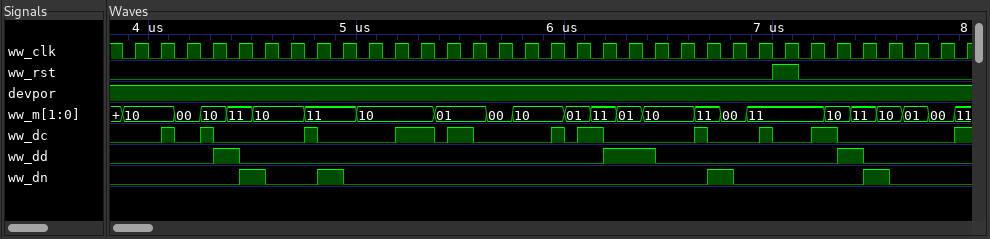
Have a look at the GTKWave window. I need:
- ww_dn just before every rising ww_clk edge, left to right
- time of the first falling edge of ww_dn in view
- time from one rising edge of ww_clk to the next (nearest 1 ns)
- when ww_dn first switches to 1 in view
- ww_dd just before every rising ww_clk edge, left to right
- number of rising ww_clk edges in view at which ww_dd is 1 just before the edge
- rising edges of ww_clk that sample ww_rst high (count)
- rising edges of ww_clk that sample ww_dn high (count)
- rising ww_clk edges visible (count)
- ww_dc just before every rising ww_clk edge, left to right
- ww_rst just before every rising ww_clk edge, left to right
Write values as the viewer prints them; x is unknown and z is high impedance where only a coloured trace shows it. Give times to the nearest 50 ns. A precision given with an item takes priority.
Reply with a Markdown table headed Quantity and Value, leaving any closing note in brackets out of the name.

| Quantity | Value |
|---|---|
| ww_dn just before every rising ww_clk edge, left to right | 0 0 0 0 0 1 0 0 1 0 0 0 0 0 0 0 0 0 0 0 0 0 0 1 0 0 0 0 0 1 0 0 0 |
| time of the first falling edge of ww_dn in view | 4550 ns |
| time from one rising edge of ww_clk to the next | 125 ns |
| when ww_dn first switches to 1 in view | 4450 ns |
| ww_dd just before every rising ww_clk edge, left to right | 0 0 0 0 1 0 0 0 0 0 0 0 0 0 0 0 0 0 0 1 1 0 0 0 0 0 0 0 1 0 0 0 0 |
| number of rising ww_clk edges in view at which ww_dd is 1 just before the edge | 4 |
| rising edges of ww_clk that sample ww_rst high | 1 |
| rising edges of ww_clk that sample ww_dn high | 4 |
| rising ww_clk edges visible | 33 |
| ww_dc just before every rising ww_clk edge, left to right | 0 0 0 1 0 0 0 1 0 0 0 1 0 1 0 0 0 0 1 0 0 0 1 0 0 0 0 1 0 0 0 0 1 |
| ww_rst just before every rising ww_clk edge, left to right | 0 0 0 0 0 0 0 0 0 0 0 0 0 0 0 0 0 0 0 0 0 0 0 0 0 1 0 0 0 0 0 0 0 |
